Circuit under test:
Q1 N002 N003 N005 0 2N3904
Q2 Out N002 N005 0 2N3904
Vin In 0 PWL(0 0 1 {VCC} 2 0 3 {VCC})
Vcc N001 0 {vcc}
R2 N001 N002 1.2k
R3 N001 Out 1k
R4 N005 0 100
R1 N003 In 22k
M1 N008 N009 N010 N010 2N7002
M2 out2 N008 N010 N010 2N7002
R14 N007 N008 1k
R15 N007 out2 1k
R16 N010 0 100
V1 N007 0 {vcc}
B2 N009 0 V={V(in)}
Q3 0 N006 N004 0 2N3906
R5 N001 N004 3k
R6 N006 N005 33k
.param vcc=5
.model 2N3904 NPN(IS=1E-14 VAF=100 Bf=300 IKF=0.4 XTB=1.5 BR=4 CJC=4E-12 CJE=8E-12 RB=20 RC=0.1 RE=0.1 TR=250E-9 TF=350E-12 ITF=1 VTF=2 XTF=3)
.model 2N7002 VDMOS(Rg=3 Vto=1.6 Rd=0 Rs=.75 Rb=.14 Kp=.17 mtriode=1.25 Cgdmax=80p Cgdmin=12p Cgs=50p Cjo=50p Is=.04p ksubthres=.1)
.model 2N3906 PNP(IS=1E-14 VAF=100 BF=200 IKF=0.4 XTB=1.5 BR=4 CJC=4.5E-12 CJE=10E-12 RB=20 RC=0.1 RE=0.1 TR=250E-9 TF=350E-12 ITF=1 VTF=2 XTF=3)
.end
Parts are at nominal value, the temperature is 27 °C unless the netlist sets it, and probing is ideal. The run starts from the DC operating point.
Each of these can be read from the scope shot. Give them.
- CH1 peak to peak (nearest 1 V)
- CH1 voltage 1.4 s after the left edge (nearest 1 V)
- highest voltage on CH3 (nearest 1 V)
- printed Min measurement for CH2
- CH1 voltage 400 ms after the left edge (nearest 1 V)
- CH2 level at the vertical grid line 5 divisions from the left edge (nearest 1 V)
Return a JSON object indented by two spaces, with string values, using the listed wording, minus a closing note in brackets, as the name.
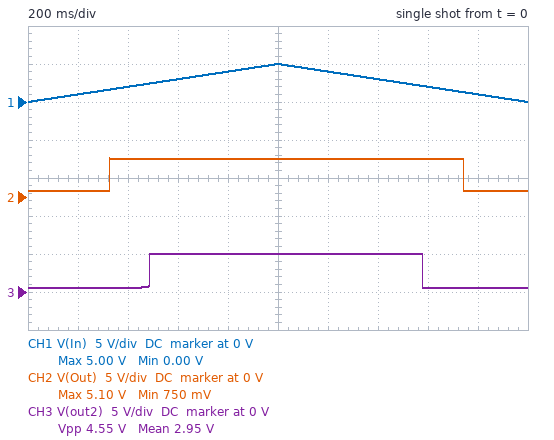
{
  "CH1 peak to peak": "5 V",
  "CH1 voltage 1.4 s after the left edge": "3 V",
  "highest voltage on CH3": "5 V",
  "printed Min measurement for CH2": "750 mV",
  "CH1 voltage 400 ms after the left edge": "2 V",
  "CH2 level at the vertical grid line 5 divisions from the left edge": "5 V"
}
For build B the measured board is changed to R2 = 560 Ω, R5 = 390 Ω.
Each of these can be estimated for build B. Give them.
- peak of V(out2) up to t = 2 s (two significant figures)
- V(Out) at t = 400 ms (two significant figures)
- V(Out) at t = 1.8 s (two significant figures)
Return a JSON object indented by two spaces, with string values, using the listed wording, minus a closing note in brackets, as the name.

{
  "peak of V(out2) up to t = 2 s": "5.0 V",
  "V(Out) at t = 400 ms": "1.0 V",
  "V(Out) at t = 1.8 s": "980 mV"
}
